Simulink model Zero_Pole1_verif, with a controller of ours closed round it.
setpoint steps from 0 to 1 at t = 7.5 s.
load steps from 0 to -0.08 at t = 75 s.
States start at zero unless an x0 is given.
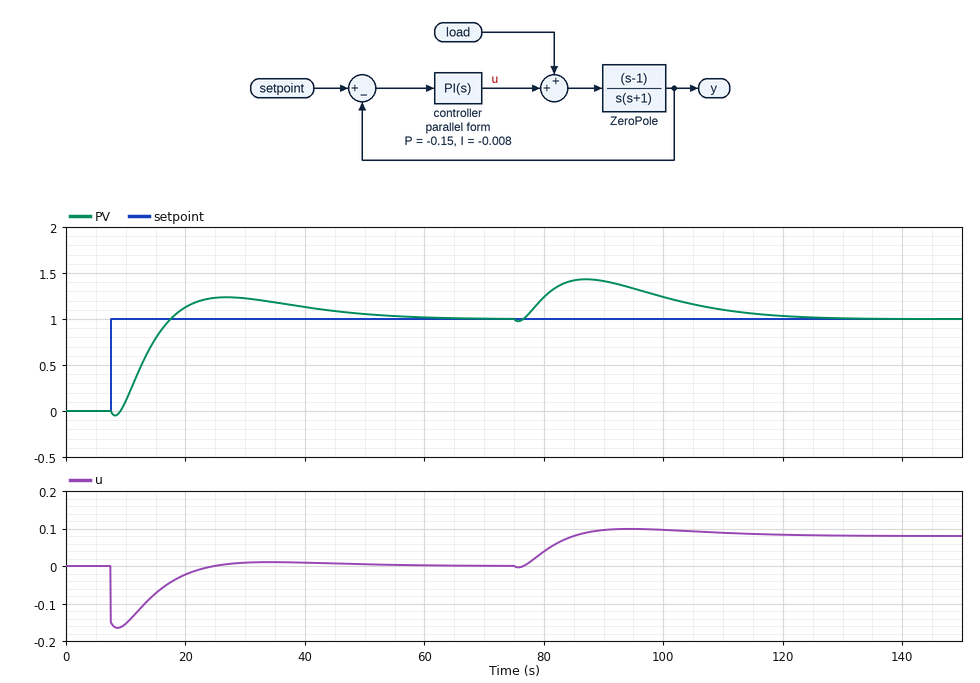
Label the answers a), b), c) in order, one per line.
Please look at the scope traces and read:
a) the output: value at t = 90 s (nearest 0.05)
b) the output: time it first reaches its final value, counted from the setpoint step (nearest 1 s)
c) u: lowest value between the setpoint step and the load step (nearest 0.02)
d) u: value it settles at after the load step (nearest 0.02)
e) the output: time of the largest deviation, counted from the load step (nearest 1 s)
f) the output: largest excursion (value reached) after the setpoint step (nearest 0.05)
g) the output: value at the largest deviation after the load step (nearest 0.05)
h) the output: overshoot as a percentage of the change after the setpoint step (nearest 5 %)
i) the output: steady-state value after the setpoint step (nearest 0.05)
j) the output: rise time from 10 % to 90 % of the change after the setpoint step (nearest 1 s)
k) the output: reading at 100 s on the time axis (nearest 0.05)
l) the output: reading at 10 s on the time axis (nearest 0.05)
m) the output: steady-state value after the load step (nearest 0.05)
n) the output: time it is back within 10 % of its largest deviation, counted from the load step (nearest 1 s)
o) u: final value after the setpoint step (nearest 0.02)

a) 1.40
b) 10 s
c) -0.16
d) 0.08
e) 12 s
f) 1.25
g) 1.45
h) 25 %
i) 1.00
j) 6 s
k) 1.25
l) 0.10
m) 1.00
n) 43 s
o) 0.00
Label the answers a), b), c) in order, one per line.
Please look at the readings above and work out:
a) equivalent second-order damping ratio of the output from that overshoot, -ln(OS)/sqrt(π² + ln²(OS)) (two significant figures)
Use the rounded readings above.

a) 0.40
